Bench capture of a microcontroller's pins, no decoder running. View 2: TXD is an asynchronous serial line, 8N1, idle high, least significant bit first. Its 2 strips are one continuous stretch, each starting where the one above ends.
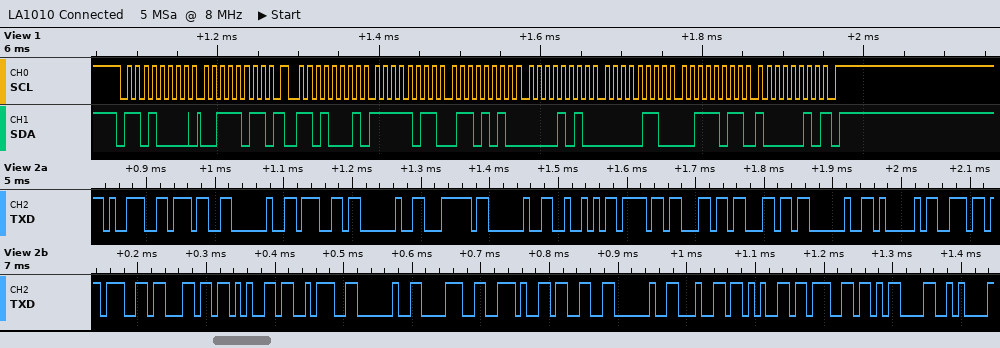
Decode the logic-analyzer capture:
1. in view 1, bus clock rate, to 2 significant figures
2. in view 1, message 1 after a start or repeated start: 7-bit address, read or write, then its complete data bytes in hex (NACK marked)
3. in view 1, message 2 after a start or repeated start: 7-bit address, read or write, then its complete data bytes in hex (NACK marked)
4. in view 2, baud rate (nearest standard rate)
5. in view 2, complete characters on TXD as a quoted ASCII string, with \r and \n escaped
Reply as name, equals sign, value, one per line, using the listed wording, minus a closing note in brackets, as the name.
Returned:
in view 1, bus clock rate, to 2 significant figures = 100 kHz
in view 1, message 1 after a start or repeated start: 7-bit address, read or write, then its complete data bytes in hex = 0x68 write: 3B
in view 1, message 2 after a start or repeated start: 7-bit address, read or write, then its complete data bytes in hex = 0x68 read: FB 6A 0A 06 3B 82 NACK
in view 2, baud rate = 115200 baud
in view 2, complete characters on TXD as a quoted ASCII string, with \r and \n escaped = "97 g | Roll Angle: 8.3 deg\r\n"
